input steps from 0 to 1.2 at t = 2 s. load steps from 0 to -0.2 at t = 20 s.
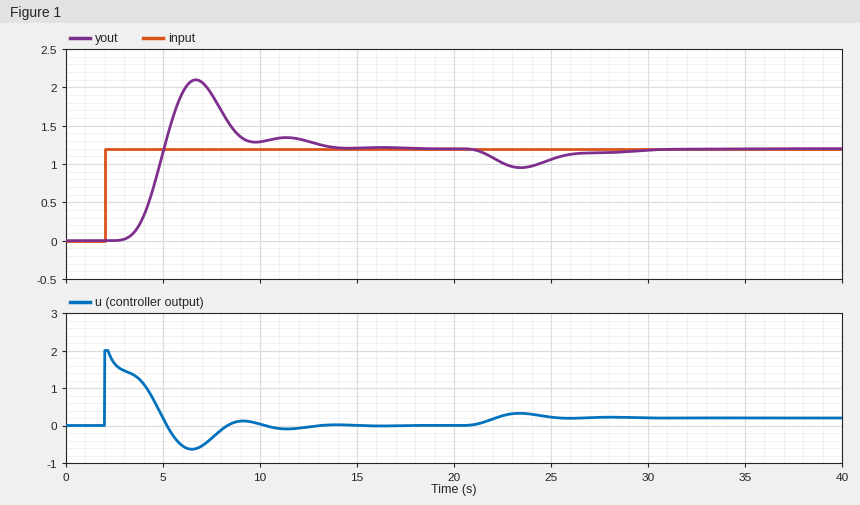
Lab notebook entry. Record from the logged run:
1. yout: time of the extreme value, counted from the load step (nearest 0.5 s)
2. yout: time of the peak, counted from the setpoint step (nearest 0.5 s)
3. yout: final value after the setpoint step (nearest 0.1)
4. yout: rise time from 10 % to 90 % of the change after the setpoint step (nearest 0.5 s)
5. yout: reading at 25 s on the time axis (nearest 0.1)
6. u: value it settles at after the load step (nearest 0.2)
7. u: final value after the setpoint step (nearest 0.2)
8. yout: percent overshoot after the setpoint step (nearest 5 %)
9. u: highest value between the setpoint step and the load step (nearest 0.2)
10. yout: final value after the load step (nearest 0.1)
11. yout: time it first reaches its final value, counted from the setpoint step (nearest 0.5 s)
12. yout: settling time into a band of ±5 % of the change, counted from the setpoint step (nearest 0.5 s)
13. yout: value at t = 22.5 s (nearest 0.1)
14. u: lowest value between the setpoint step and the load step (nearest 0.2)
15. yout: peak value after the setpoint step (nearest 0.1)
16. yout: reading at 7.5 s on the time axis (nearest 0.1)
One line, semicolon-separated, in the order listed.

3.5 s; 4.5 s; 1.2; 1.5 s; 1.1; 0.2; 0.0; 75 %; 2.0; 1.2; 3.0 s; 11.0 s; 1.0; -0.6; 2.1; 1.9
